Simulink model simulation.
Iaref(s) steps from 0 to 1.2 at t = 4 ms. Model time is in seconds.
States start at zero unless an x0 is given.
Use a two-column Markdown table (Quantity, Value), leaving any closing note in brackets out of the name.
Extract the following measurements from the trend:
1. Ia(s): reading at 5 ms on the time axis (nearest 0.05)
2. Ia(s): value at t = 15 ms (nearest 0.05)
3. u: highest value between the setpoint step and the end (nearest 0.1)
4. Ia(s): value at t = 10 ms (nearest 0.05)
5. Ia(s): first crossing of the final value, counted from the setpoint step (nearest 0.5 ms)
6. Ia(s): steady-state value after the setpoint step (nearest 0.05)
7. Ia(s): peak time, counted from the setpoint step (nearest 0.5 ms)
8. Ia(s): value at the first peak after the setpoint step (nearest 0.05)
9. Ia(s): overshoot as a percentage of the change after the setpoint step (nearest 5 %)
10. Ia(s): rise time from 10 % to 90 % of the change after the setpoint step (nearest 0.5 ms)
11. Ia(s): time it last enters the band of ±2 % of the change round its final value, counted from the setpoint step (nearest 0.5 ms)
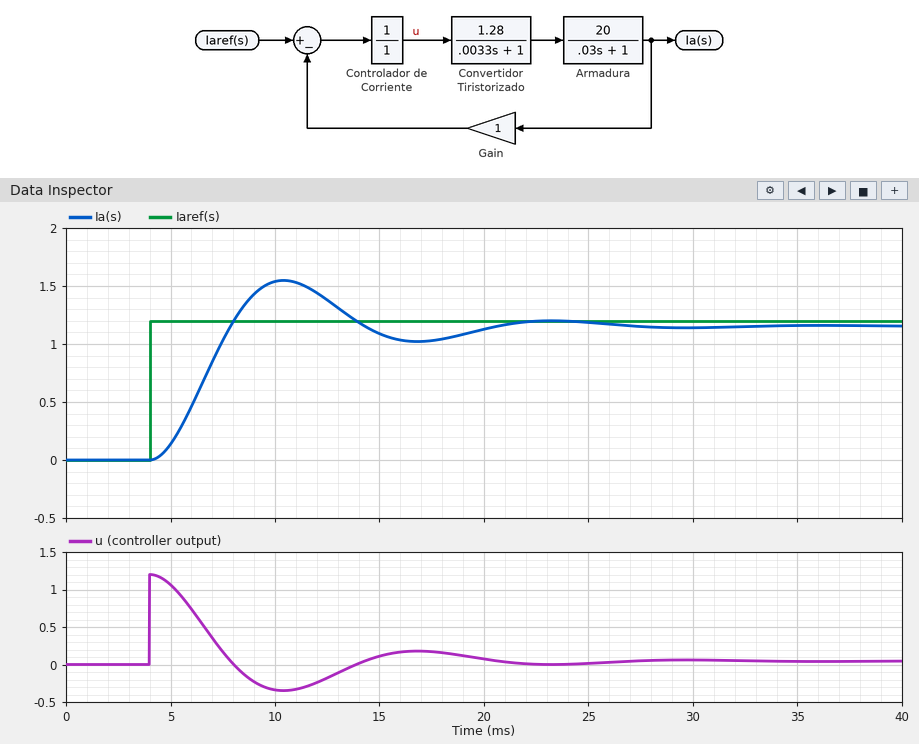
| Quantity | Value |
|---|---|
| Ia(s): reading at 5 ms on the time axis | 0.15 |
| Ia(s): value at t = 15 ms | 1.10 |
| u: highest value between the setpoint step and the end | 1.2 |
| Ia(s): value at t = 10 ms | 1.55 |
| Ia(s): first crossing of the final value, counted from the setpoint step | 4.0 ms |
| Ia(s): steady-state value after the setpoint step | 1.15 |
| Ia(s): peak time, counted from the setpoint step | 6.5 ms |
| Ia(s): value at the first peak after the setpoint step | 1.55 |
| Ia(s): overshoot as a percentage of the change after the setpoint step | 35 % |
| Ia(s): rise time from 10 % to 90 % of the change after the setpoint step | 2.5 ms |
| Ia(s): time it last enters the band of ±2 % of the change round its final value, counted from the setpoint step | 21.5 ms |
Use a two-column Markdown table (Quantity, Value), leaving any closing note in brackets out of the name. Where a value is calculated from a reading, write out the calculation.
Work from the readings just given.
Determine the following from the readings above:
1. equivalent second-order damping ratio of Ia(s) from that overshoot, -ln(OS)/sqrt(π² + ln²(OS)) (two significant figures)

| Quantity | Value |
|---|---|
| equivalent second-order damping ratio of Ia(s) from that overshoot, -ln(OS)/sqrt(π² + ln²(OS)) | ln(0.35) = -1.050; 1.050 / sqrt(9.870 + 1.102) = 0.32 |
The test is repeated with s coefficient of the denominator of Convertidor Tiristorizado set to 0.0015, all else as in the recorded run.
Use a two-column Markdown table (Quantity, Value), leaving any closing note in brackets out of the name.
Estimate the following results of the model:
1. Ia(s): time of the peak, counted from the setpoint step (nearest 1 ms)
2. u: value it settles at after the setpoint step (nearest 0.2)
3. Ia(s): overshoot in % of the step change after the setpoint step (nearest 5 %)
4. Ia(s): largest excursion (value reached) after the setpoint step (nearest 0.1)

| Quantity | Value |
|---|---|
| Ia(s): time of the peak, counted from the setpoint step | 5 ms |
| u: value it settles at after the setpoint step | 0.0 |
| Ia(s): overshoot in % of the step change after the setpoint step | 20 % |
| Ia(s): largest excursion (value reached) after the setpoint step | 1.4 |
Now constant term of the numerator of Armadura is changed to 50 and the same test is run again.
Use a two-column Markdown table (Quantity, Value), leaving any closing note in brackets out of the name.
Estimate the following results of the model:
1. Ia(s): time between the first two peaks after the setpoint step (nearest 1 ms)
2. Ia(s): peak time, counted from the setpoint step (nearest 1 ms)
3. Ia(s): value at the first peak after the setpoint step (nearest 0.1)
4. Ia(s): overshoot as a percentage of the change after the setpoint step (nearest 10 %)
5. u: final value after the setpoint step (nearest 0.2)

| Quantity | Value |
|---|---|
| Ia(s): time between the first two peaks after the setpoint step | 8 ms |
| Ia(s): peak time, counted from the setpoint step | 4 ms |
| Ia(s): value at the first peak after the setpoint step | 1.8 |
| Ia(s): overshoot as a percentage of the change after the setpoint step | 50 % |
| u: final value after the setpoint step | 0.0 |
